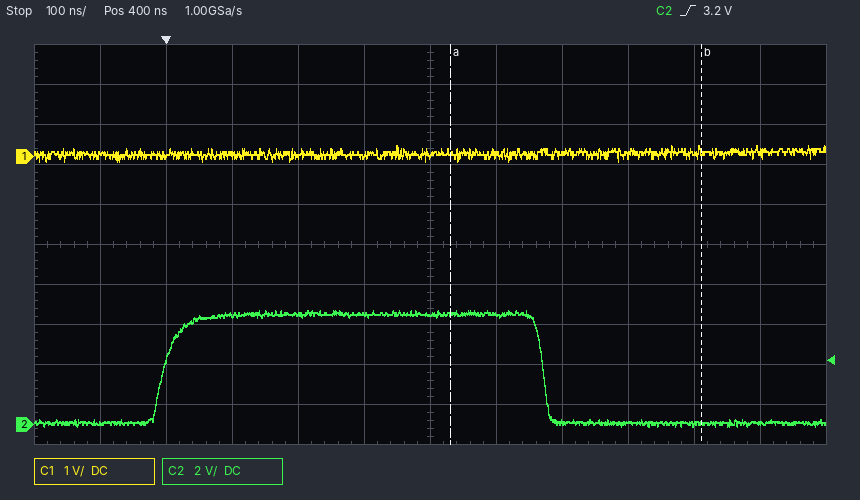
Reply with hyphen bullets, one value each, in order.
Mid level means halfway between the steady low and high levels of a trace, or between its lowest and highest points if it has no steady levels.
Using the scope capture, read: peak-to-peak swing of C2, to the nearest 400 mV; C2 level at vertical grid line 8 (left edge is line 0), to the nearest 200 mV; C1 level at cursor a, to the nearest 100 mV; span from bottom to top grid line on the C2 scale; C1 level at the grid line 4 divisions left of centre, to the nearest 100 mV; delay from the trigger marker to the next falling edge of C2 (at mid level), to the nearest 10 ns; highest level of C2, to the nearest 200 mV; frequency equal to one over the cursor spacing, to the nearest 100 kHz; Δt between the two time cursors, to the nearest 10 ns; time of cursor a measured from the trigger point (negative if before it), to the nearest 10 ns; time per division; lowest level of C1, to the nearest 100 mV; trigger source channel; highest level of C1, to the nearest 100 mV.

- 5.6 V
- 200 mV
- 100 mV
- 20 V
- 0.0 V
- 570 ns
- 5.6 V
- 2.6 MHz
- 380 ns
- +430 ns
- 100 ns
- -100 mV
- C2
- 300 mV
